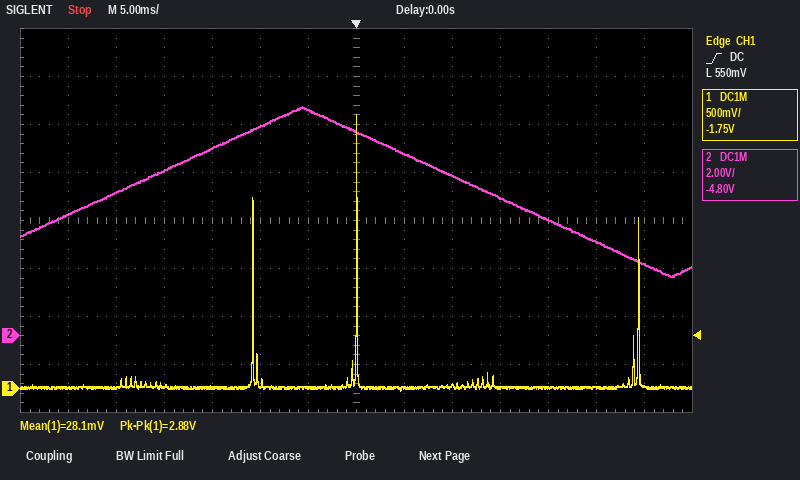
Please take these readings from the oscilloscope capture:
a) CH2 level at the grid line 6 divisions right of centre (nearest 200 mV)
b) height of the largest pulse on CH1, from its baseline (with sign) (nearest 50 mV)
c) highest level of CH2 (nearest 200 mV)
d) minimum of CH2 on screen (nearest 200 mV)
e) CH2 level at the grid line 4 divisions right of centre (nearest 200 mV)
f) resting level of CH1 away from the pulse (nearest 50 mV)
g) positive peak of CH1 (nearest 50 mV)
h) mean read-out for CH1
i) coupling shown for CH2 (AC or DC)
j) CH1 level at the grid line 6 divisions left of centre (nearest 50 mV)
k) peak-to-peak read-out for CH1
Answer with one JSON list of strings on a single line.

["3.0 V", "+2.85 V", "9.6 V", "2.4 V", "4.8 V", "0 mV", "2.85 V", "28.1 mV", "DC", "0 mV", "2.88 V"]
